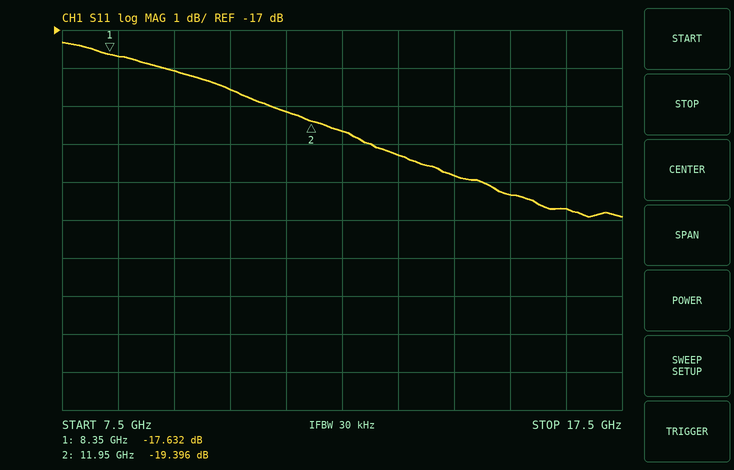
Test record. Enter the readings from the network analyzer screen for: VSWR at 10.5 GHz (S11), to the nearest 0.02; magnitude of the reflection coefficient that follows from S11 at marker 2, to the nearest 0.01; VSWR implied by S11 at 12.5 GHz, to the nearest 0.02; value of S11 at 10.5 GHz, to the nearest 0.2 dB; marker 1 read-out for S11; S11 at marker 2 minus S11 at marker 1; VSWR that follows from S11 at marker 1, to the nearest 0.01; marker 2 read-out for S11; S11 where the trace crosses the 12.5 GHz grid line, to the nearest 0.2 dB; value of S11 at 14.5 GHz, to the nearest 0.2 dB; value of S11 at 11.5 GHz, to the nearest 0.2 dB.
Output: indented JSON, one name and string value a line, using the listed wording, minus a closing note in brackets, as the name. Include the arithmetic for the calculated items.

{
  "VSWR at 10.5 GHz (S11), to the nearest 0.02": "|Γ| = 10^(-18.6/20) = 0.1175; VSWR = (1 + 0.1175)/(1 − 0.1175) ≈ 1.27, so 1.26 to the nearest 0.02",
  "magnitude of the reflection coefficient that follows from S11 at marker 2, to the nearest 0.01": "10^(-19.396/20) ≈ 0.11",
  "VSWR implied by S11 at 12.5 GHz, to the nearest 0.02": "|Γ| = 10^(-19.6/20) = 0.1047; VSWR = (1 + 0.1047)/(1 − 0.1047) ≈ 1.23, so 1.24 to the nearest 0.02",
  "value of S11 at 10.5 GHz, to the nearest 0.2 dB": "-18.6 dB",
  "marker 1 read-out for S11": "-17.632 dB",
  "S11 at marker 2 minus S11 at marker 1": "-19.396 − (-17.632) = -1.764 dB",
  "VSWR that follows from S11 at marker 1, to the nearest 0.01": "(1 + 0.1313)/(1 − 0.1313) ≈ 1.30",
  "marker 2 read-out for S11": "-19.396 dB",
  "S11 where the trace crosses the 12.5 GHz grid line, to the nearest 0.2 dB": "-19.6 dB",
  "value of S11 at 14.5 GHz, to the nearest 0.2 dB": "-20.8 dB",
  "value of S11 at 11.5 GHz, to the nearest 0.2 dB": "-19.2 dB"
}
